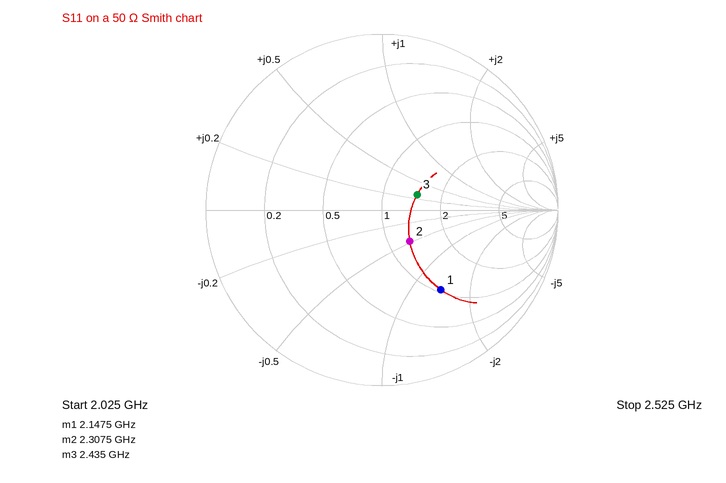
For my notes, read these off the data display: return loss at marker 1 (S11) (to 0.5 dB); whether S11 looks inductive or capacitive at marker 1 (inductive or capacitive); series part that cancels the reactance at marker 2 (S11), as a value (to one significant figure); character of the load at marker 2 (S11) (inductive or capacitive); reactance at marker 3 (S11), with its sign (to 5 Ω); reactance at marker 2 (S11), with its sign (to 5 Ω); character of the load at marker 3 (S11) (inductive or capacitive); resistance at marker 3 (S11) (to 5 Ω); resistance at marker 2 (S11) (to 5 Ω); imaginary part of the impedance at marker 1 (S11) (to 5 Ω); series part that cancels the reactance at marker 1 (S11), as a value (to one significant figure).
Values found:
5.0 dB
capacitive
2 nH
capacitive
+15 Ω
-25 Ω
inductive
75 Ω
65 Ω
-70 Ω
5 nH
